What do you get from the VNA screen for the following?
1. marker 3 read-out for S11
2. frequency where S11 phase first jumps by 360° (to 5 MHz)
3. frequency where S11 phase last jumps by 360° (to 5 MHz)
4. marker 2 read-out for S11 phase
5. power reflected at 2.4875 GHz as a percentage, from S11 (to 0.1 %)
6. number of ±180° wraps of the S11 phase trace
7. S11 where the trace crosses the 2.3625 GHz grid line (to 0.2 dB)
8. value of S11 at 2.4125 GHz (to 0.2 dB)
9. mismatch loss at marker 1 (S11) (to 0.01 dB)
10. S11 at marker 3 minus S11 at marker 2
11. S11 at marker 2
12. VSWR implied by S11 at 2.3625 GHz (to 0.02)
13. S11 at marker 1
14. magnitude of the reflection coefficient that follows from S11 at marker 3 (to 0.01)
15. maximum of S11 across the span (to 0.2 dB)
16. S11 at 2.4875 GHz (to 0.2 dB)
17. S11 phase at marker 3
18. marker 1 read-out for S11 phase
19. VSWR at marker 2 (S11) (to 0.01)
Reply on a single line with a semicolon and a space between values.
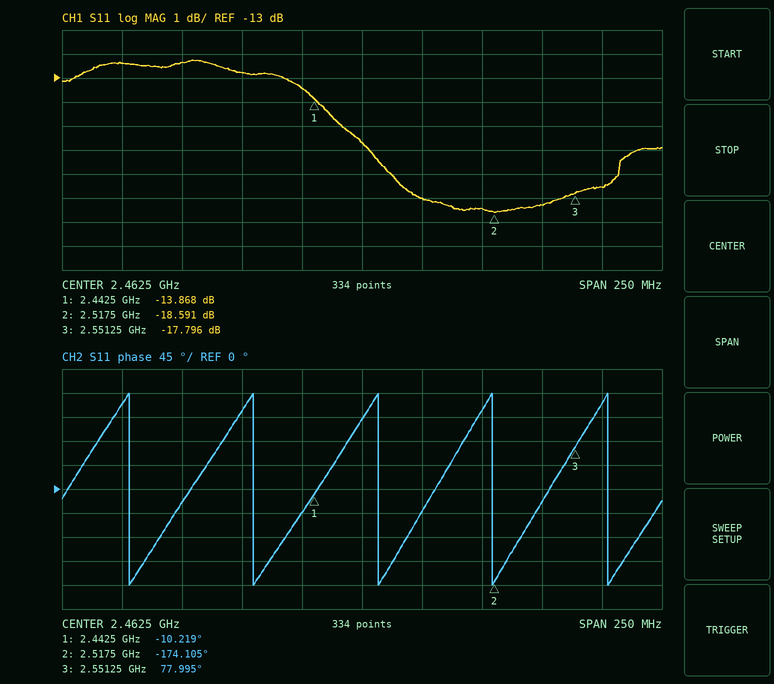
-17.796 dB; 2.365 GHz; 2.565 GHz; -174.105°; 1.6 %; 5; -12.4 dB; -12.8 dB; 0.18 dB; 0.795 dB; -18.591 dB; 1.64; -13.868 dB; 0.13; -12.2 dB; -18.0 dB; 77.995°; -10.219°; 1.27
